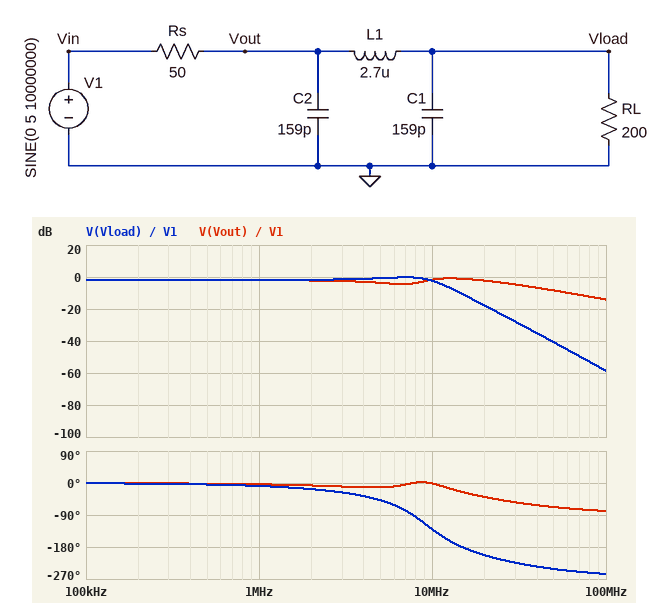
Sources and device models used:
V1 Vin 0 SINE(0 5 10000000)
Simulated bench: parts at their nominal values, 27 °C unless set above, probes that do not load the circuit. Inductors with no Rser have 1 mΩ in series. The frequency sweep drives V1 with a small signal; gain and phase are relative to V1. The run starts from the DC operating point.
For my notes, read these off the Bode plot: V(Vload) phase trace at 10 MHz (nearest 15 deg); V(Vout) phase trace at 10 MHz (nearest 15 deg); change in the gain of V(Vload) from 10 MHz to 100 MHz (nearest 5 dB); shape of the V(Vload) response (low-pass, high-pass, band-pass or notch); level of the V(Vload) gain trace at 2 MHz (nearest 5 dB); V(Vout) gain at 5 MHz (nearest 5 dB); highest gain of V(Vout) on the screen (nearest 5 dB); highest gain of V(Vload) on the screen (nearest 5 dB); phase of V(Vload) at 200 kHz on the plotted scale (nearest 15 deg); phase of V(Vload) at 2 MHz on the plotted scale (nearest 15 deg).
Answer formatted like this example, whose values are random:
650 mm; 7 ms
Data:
-135 deg; 0 deg; -55 dB; low-pass; 0 dB; -5 dB; 0 dB; 0 dB; 0 deg; -15 deg
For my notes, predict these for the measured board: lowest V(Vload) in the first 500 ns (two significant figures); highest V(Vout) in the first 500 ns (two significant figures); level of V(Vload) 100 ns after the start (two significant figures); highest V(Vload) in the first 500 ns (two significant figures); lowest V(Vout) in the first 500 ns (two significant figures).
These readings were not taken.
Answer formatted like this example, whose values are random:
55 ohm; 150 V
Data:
-3.8 V; 4.1 V; -3.1 V; 3.8 V; -4.1 V
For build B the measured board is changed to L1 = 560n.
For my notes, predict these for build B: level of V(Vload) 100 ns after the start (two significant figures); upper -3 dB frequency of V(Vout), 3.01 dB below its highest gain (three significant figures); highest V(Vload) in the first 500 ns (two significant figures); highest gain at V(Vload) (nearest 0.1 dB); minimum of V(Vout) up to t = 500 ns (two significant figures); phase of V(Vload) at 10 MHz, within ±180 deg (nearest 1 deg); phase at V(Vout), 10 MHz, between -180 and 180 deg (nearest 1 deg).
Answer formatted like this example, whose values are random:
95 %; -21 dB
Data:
-3.0 V; 36.4 MHz; 4.1 V; -0.6 dB; -2.7 V; -51 deg; -36 deg
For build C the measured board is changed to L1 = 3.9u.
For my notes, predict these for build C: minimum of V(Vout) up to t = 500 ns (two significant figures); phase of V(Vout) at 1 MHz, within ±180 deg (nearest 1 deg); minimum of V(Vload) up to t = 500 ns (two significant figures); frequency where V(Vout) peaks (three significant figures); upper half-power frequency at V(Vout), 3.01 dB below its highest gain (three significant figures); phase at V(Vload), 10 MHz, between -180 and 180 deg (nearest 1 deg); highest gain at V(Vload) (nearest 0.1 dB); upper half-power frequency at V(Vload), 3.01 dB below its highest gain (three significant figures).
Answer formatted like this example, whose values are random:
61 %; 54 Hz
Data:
-4.6 V; -3 deg; -2.8 V; 10.7 MHz; 25.0 MHz; -151 deg; -0.6 dB; 8.57 MHz
